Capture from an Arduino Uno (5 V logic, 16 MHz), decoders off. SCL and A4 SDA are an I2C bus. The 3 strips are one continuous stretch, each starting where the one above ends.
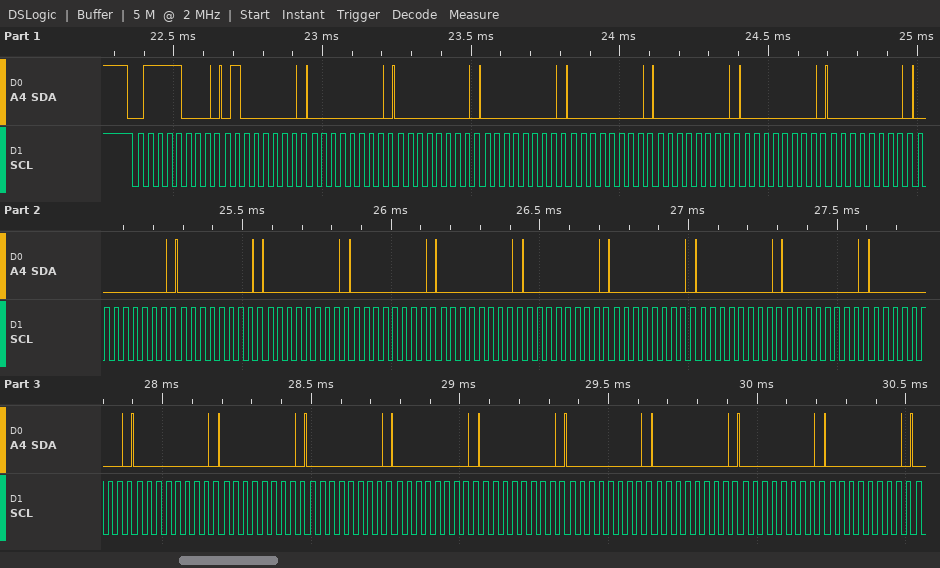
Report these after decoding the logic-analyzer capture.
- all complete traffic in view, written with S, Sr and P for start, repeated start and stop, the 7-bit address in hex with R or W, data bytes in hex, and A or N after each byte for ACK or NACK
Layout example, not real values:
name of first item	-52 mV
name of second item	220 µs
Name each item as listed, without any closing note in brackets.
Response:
all complete traffic in view, written with S, Sr and P for start, repeated start and stop, the 7-bit address in hex with R or W, data bytes in hex, and A or N after each byte for ACK or NACK	S 3CW A 40 A 00 A 00 A 00 A 00 A 00 A 00 A 00 A 00 A 00 A 00 A 00 A 00 A 00 A 00 A 00 A 00 A 00 A 00 A 00 A 00 A 00 A 00 A 00 A 00 A 00 A 00 A
